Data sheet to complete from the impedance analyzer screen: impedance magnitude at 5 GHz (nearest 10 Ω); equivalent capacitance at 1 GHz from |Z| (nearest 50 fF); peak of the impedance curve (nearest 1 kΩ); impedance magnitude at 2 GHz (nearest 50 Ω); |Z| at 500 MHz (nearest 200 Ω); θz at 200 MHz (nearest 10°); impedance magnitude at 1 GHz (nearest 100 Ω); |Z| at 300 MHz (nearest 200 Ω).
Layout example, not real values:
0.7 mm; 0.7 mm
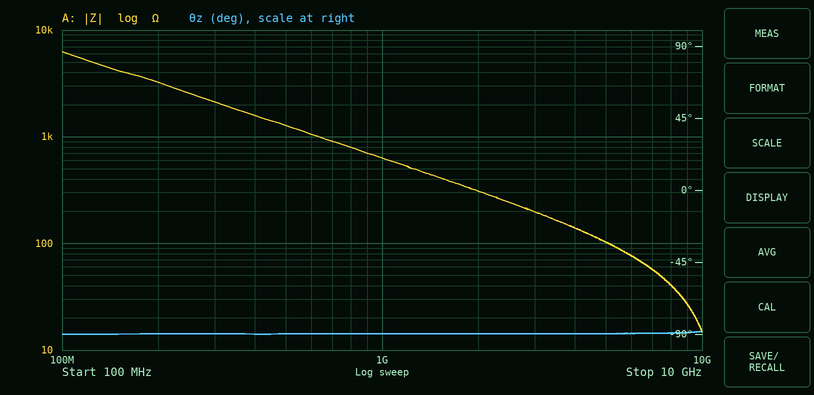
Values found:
100 Ω; 250 fF; 6 kΩ; 300 Ω; 1.2 kΩ; -90°; 600 Ω; 2.2 kΩ
